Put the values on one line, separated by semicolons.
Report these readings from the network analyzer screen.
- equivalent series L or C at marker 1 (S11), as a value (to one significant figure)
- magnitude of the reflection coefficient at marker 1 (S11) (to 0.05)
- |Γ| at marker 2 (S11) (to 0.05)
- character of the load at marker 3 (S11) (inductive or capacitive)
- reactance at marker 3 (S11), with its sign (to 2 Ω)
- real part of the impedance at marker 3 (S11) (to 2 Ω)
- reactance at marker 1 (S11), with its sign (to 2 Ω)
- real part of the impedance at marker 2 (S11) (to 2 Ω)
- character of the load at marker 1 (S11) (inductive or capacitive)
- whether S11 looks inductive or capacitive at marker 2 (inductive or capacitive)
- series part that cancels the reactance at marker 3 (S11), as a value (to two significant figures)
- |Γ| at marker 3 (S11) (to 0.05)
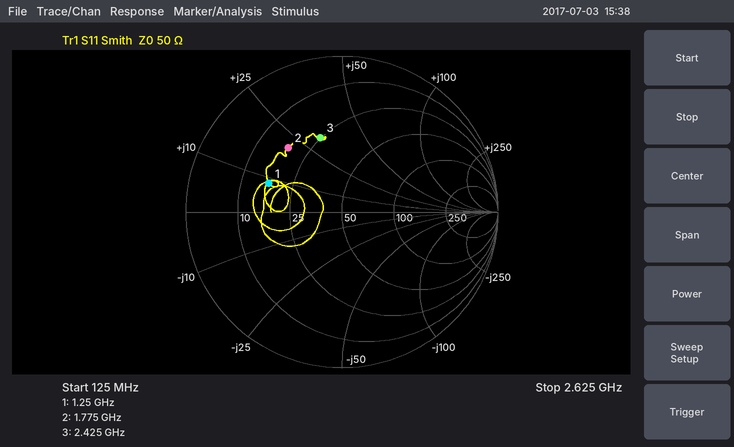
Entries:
1 nH; 0.50; 0.55; inductive; +32 Ω; 24 Ω; +8 Ω; 18 Ω; inductive; inductive; 2.1 pF; 0.50
